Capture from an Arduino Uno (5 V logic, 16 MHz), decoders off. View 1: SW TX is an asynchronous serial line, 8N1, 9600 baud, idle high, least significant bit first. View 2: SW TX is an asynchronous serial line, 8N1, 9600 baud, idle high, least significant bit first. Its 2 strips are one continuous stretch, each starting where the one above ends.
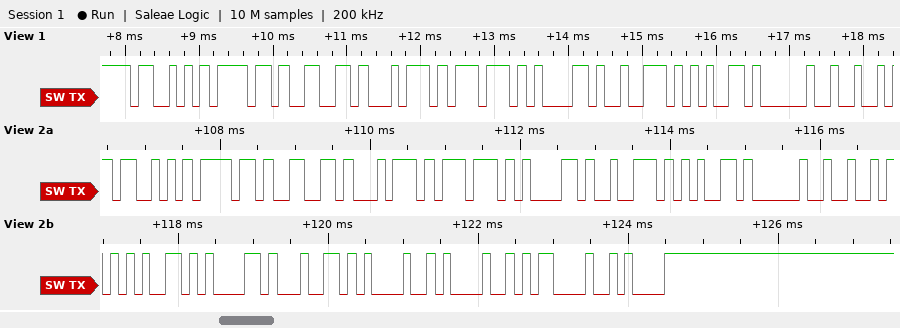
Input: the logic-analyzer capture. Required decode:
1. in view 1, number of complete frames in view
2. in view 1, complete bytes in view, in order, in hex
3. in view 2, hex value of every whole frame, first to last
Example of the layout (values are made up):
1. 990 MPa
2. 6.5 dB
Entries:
1. 9
2. 53 6F 66 74 77 61 72 65 20
3. 53 6F 66 74 77 61 72 65 20 52 65 61 64 21 21 0D 0A
